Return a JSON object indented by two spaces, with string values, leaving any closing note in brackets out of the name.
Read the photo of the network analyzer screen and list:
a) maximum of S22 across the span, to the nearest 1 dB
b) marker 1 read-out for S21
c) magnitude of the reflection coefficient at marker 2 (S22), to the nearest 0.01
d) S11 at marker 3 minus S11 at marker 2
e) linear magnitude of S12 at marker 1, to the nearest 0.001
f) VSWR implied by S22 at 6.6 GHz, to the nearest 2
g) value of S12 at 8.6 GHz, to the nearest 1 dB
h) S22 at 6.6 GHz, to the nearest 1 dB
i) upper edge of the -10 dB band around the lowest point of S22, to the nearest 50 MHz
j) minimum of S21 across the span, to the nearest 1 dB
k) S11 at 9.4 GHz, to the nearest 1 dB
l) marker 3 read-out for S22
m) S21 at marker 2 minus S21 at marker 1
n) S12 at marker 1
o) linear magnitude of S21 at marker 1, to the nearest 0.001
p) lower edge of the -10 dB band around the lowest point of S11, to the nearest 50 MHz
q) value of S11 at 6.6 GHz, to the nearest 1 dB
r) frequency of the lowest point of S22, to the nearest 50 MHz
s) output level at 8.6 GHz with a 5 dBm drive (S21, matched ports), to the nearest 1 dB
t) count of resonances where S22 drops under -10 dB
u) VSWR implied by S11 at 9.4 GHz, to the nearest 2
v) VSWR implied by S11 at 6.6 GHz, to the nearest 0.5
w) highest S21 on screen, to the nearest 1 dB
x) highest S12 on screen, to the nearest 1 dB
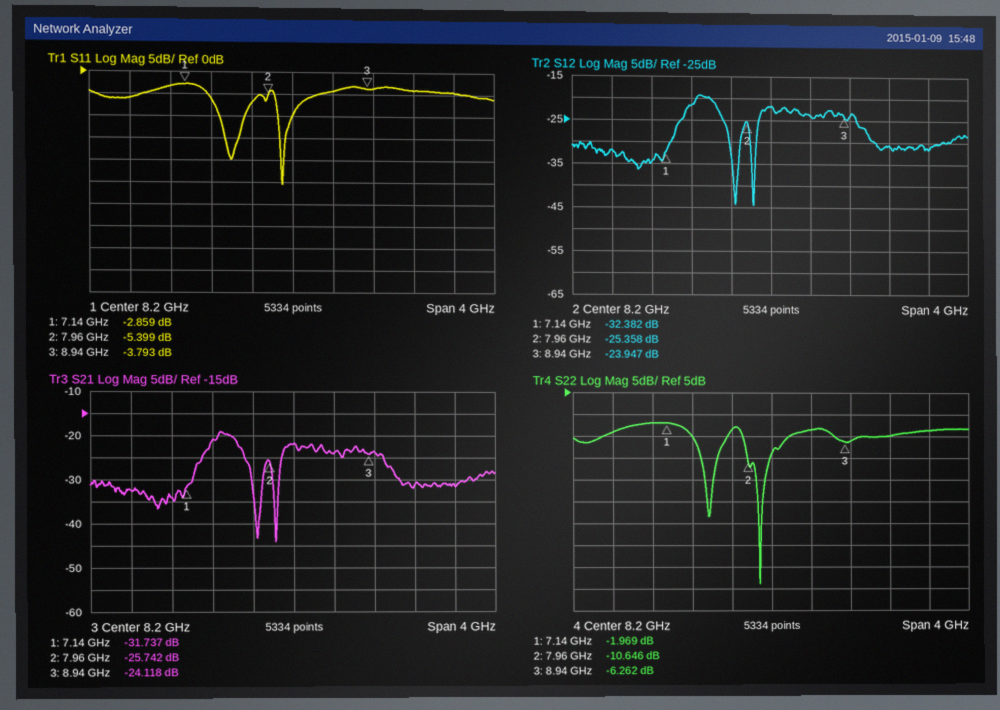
{
  "maximum of S22 across the span, to the nearest 1 dB": "-2 dB",
  "marker 1 read-out for S21": "-31.737 dB",
  "magnitude of the reflection coefficient at marker 2 (S22), to the nearest 0.01": "0.29",
  "S11 at marker 3 minus S11 at marker 2": "1.606 dB",
  "linear magnitude of S12 at marker 1, to the nearest 0.001": "0.024",
  "VSWR implied by S22 at 6.6 GHz, to the nearest 2": "4",
  "value of S12 at 8.6 GHz, to the nearest 1 dB": "-24 dB",
  "S22 at 6.6 GHz, to the nearest 1 dB": "-4 dB",
  "upper edge of the -10 dB band around the lowest point of S22, to the nearest 50 MHz": "8.20 GHz",
  "minimum of S21 across the span, to the nearest 1 dB": "-44 dB",
  "S11 at 9.4 GHz, to the nearest 1 dB": "-4 dB",
  "marker 3 read-out for S22": "-6.262 dB",
  "S21 at marker 2 minus S21 at marker 1": "5.995 dB",
  "S12 at marker 1": "-32.382 dB",
  "linear magnitude of S21 at marker 1, to the nearest 0.001": "0.026",
  "lower edge of the -10 dB band around the lowest point of S11, to the nearest 50 MHz": "8.05 GHz",
  "value of S11 at 6.6 GHz, to the nearest 1 dB": "-6 dB",
  "frequency of the lowest point of S22, to the nearest 50 MHz": "8.10 GHz",
  "output level at 8.6 GHz with a 5 dBm drive (S21, matched ports), to the nearest 1 dB": "-19 dBm",
  "count of resonances where S22 drops under -10 dB": "2",
  "VSWR implied by S11 at 9.4 GHz, to the nearest 2": "4",
  "VSWR implied by S11 at 6.6 GHz, to the nearest 0.5": "3.0",
  "highest S21 on screen, to the nearest 1 dB": "-19 dB",
  "highest S12 on screen, to the nearest 1 dB": "-19 dB"
}
